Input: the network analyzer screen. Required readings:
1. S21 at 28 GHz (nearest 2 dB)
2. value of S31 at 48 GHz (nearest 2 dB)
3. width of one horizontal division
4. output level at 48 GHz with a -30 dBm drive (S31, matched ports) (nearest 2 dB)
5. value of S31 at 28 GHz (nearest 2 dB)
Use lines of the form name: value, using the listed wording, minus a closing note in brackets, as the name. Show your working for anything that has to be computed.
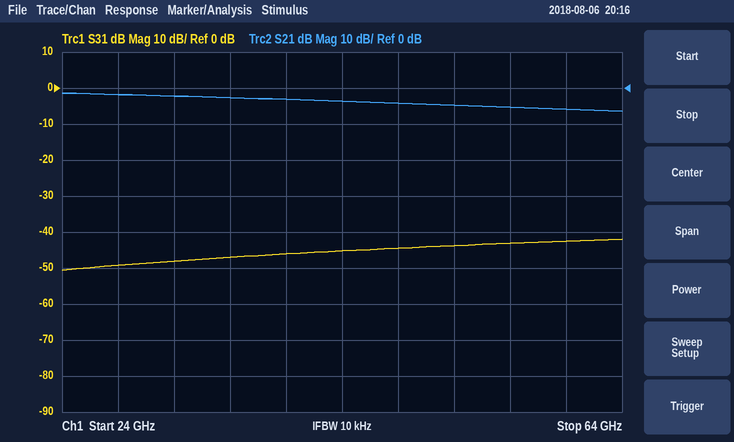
S21 at 28 GHz: -2 dB
value of S31 at 48 GHz: -44 dB
width of one horizontal division: 4 GHz
output level at 48 GHz with a -30 dBm drive (S31, matched ports): -30 dBm + (-44 dB) = -74 dBm
value of S31 at 28 GHz: -50 dB
